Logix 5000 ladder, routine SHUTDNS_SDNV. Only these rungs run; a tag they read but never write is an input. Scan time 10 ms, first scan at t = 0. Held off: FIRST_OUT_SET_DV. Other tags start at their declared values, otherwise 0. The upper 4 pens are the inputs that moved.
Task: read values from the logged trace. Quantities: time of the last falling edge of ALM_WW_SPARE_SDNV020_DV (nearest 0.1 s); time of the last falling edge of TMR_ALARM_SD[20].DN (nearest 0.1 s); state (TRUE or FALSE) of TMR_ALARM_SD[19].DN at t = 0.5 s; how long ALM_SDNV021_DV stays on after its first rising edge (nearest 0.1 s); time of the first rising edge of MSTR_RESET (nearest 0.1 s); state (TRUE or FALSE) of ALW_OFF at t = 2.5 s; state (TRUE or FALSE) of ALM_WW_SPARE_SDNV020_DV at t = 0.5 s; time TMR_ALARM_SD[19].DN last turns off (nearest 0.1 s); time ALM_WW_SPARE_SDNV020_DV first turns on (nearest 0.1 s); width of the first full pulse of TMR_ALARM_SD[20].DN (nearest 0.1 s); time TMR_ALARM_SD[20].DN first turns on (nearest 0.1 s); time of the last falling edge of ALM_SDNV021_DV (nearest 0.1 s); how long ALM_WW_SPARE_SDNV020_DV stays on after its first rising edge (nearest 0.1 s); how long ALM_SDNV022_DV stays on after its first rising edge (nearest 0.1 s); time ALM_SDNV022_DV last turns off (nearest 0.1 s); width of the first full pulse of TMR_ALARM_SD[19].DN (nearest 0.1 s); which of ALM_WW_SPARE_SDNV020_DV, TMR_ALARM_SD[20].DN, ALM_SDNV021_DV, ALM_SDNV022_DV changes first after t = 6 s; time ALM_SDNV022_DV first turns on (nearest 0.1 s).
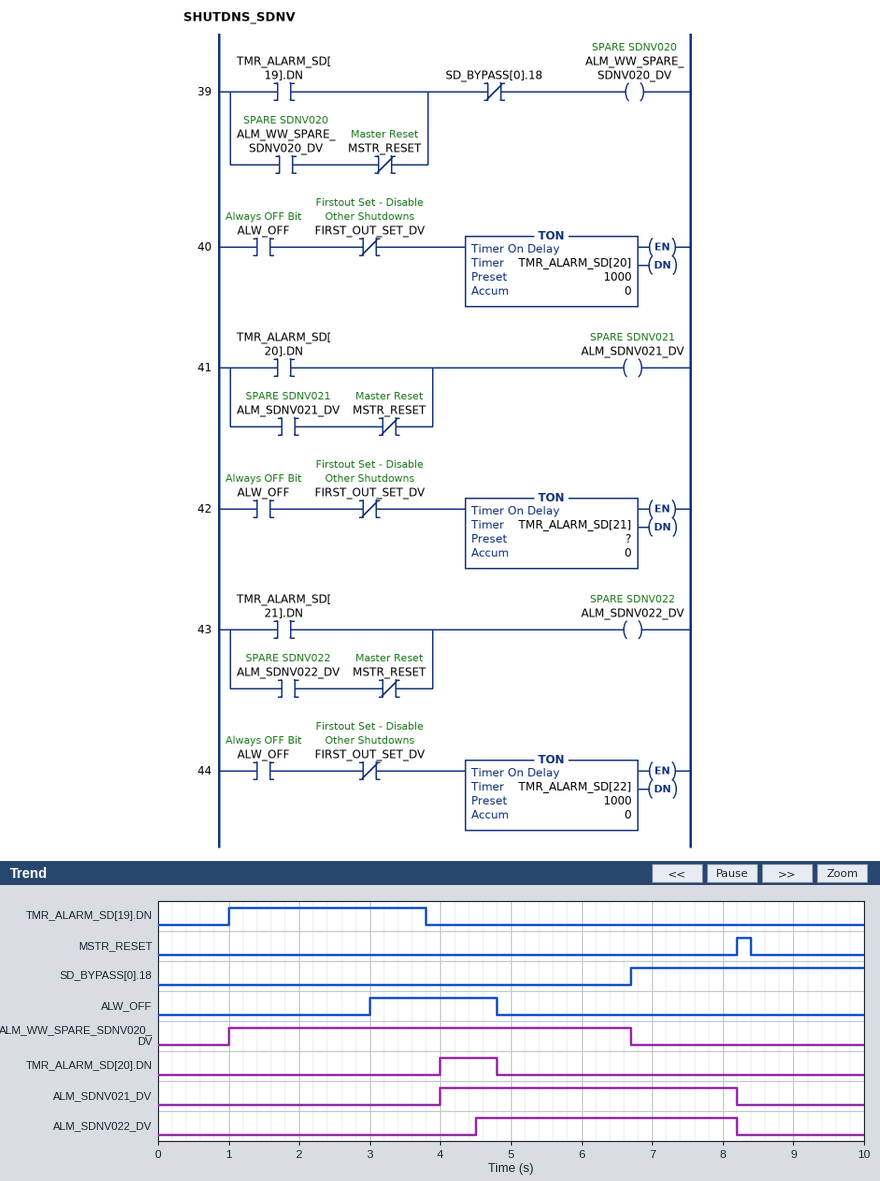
6.7 s
4.8 s
FALSE
4.2 s
8.2 s
FALSE
FALSE
3.8 s
1.0 s
0.8 s
4.0 s
8.2 s
5.7 s
3.7 s
8.2 s
2.8 s
ALM_WW_SPARE_SDNV020_DV
4.5 s
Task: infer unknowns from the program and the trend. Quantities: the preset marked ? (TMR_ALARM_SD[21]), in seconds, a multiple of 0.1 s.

1.5 s
